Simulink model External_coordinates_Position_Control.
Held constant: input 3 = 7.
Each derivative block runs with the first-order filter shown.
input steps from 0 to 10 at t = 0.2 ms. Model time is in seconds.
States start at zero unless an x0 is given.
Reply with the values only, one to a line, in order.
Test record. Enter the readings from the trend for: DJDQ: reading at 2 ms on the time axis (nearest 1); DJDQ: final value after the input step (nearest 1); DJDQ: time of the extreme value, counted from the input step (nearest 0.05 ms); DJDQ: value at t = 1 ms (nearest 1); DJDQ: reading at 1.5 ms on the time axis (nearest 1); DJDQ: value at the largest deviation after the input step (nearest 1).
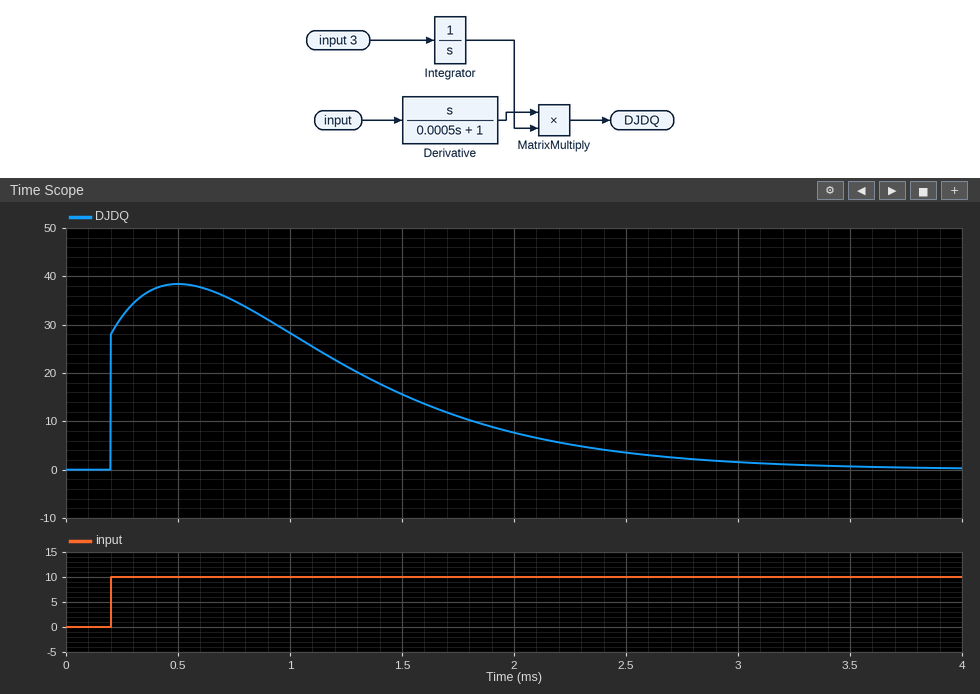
8
0
0.30 ms
28
16
38
